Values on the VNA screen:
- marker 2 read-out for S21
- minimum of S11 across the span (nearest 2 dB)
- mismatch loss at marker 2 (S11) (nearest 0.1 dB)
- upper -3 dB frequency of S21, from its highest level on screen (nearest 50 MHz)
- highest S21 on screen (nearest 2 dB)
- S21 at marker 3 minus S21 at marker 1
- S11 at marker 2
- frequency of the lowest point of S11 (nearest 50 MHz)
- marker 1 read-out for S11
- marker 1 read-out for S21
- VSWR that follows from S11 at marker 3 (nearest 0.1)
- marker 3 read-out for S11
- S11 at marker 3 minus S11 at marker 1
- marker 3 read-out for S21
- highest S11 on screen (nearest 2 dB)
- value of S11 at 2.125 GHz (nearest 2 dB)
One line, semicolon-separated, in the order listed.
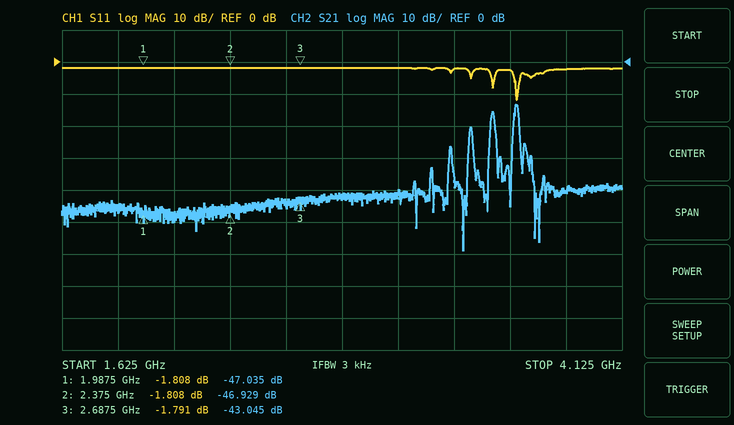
-46.929 dB; -12 dB; 4.7 dB; 3.65 GHz; -14 dB; 3.990 dB; -1.808 dB; 3.65 GHz; -1.808 dB; -47.035 dB; 9.7; -1.791 dB; 0.017 dB; -43.045 dB; -2 dB; -2 dB
